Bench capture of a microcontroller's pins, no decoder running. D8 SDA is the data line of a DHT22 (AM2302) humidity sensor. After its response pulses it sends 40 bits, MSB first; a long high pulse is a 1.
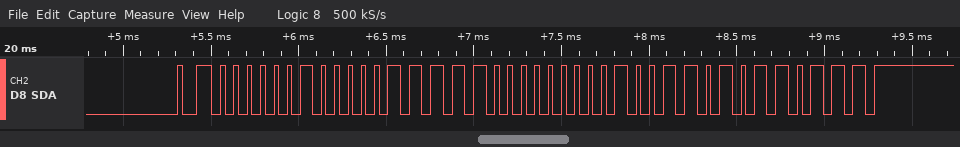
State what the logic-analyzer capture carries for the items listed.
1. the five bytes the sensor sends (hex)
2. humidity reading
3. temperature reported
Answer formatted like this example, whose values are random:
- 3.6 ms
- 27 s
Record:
- 02 0F 80 26 B7
- 52.7 %
- -3.8 °C
